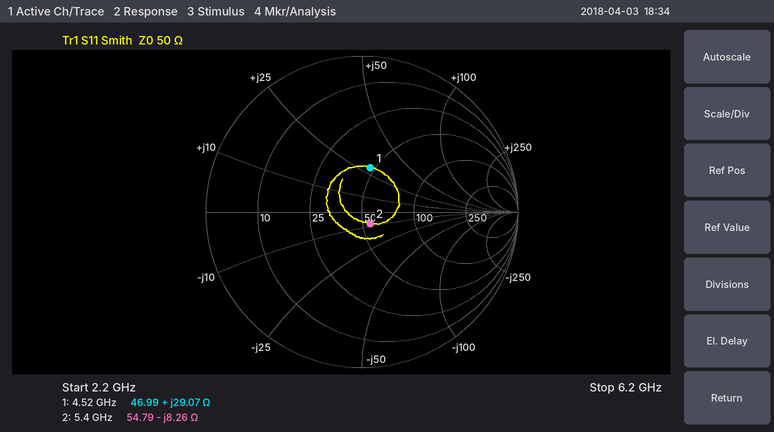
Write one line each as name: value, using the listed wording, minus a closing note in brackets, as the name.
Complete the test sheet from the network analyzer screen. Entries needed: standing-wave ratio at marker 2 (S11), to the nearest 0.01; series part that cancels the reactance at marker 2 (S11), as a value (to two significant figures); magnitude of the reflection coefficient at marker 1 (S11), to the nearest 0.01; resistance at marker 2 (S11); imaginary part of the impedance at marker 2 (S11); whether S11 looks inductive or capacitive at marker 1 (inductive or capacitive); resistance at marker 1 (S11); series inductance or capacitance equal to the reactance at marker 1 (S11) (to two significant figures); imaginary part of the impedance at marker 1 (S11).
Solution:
standing-wave ratio at marker 2 (S11), to the nearest 0.01: 1.20
series part that cancels the reactance at marker 2 (S11), as a value: 240 pH
magnitude of the reflection coefficient at marker 1 (S11), to the nearest 0.01: 0.29
resistance at marker 2: 54.79 Ω
imaginary part of the impedance at marker 2: -8.26 Ω
whether S11 looks inductive or capacitive at marker 1: inductive
resistance at marker 1: 46.99 Ω
series inductance or capacitance equal to the reactance at marker 1 (S11): 1.0 nH
imaginary part of the impedance at marker 1: +29.07 Ω
